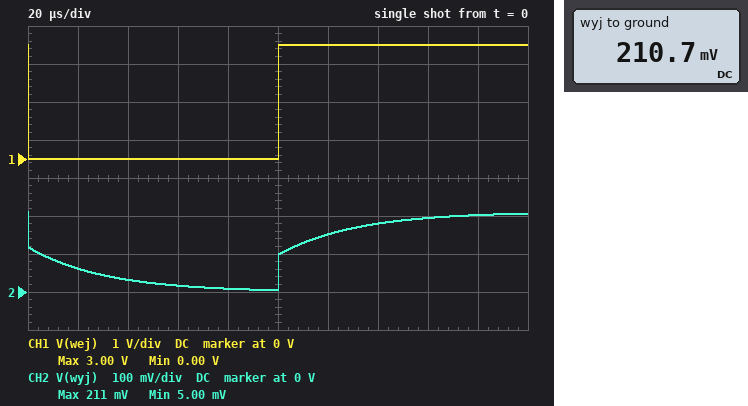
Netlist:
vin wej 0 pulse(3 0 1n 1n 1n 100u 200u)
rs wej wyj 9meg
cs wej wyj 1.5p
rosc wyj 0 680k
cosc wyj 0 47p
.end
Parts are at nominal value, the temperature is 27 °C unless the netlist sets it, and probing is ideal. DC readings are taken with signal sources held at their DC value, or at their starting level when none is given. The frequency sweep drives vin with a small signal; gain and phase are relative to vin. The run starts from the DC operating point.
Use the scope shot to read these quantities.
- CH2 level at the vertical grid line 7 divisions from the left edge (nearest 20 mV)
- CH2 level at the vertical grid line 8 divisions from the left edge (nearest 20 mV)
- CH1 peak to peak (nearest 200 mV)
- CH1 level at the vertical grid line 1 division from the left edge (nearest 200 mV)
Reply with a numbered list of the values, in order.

1. 180 mV
2. 200 mV
3. 3.0 V
4. 0 V
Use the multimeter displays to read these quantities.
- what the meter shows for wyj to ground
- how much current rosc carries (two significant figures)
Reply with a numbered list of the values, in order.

1. 210.7 mV
2. 310 nA
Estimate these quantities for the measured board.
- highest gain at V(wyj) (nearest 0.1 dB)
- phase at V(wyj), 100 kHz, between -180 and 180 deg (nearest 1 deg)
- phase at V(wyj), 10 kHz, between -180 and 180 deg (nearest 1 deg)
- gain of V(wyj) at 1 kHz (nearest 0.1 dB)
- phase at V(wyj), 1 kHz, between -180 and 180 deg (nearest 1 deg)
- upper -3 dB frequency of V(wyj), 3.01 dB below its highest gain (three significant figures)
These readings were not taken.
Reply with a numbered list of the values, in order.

1. -23.1 dB
2. -4 deg
3. -22 deg
4. -23.2 dB
5. -6 deg
6. 6.63 kHz
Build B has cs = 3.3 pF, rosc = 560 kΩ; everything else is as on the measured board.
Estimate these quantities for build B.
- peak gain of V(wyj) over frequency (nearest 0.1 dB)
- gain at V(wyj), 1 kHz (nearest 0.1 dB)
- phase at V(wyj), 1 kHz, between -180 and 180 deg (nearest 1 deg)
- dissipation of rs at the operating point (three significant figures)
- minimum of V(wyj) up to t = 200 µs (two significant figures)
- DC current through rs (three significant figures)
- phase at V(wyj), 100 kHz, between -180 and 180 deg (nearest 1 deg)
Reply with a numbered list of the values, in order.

1. -23.7 dB
2. -24.6 dB
3. 1 deg
4. 886 nW
5. -21 mV
6. 314 nA
7. 0 deg
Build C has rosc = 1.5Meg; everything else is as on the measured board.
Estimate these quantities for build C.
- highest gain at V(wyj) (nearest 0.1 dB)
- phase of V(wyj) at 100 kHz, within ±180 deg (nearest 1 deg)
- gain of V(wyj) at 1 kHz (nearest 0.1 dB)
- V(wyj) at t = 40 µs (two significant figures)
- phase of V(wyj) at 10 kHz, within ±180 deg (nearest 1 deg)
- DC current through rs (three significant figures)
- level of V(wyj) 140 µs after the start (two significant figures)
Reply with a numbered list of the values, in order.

1. -16.9 dB
2. -5 deg
3. -17.5 dB
4. 180 mV
5. -35 deg
6. 286 nA
7. 290 mV
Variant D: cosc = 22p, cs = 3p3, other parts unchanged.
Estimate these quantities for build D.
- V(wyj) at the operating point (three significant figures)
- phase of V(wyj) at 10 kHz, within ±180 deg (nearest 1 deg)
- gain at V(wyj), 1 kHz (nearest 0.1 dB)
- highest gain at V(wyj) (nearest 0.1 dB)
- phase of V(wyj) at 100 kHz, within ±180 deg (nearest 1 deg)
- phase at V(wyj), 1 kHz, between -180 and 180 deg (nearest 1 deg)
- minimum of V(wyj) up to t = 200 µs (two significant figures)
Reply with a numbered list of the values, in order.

1. 211 mV
2. 17 deg
3. -23.0 dB
4. -17.7 dB
5. 3 deg
6. 5 deg
7. -180 mV
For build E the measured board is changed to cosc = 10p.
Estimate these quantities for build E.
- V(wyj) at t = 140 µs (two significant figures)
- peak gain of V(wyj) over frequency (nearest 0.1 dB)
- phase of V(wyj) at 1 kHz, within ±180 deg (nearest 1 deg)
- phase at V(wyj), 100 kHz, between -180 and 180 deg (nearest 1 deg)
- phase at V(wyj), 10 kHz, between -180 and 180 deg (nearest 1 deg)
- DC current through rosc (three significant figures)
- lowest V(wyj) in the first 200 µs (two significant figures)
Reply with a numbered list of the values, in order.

1. 210 mV
2. -17.7 dB
3. 2 deg
4. 6 deg
5. 16 deg
6. 310 nA
7. -180 mV
